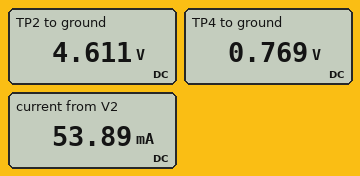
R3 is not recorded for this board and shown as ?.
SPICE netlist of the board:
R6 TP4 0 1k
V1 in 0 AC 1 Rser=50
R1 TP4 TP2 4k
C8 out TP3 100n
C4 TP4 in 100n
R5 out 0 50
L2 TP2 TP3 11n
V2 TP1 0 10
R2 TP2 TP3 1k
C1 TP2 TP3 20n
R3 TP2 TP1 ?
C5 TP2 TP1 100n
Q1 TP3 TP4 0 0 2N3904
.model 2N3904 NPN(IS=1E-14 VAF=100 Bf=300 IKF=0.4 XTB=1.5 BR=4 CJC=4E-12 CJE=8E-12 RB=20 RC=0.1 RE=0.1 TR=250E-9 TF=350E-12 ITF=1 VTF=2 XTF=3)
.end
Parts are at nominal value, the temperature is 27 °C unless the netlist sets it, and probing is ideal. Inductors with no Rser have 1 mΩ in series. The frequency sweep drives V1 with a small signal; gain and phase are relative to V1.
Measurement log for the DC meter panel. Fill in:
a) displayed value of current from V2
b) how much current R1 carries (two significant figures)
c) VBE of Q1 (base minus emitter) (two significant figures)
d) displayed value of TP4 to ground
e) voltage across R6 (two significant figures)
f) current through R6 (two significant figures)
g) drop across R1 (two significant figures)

53.89 mA
960 µA
770 mV
0.769 V
770 mV
770 µA
3.8 V
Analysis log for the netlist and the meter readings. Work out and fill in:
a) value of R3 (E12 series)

100 Ω
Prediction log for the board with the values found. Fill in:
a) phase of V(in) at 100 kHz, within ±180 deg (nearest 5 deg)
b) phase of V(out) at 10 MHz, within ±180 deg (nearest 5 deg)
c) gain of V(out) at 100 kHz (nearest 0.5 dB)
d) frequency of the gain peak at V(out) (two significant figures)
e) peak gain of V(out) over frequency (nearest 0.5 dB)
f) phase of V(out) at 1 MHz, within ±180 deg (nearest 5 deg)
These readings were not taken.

5 deg
-155 deg
22.0 dB
11 MHz
25.0 dB
85 deg
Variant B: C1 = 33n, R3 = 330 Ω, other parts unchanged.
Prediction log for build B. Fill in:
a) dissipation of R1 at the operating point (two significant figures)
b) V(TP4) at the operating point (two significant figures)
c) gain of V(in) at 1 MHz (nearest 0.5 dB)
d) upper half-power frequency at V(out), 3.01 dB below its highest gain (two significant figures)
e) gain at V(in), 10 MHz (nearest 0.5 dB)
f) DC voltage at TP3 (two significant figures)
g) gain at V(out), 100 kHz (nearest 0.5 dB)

2.5 mW
730 mV
-1.5 dB
8.4 MHz
-3.5 dB
3.9 V
16.5 dB
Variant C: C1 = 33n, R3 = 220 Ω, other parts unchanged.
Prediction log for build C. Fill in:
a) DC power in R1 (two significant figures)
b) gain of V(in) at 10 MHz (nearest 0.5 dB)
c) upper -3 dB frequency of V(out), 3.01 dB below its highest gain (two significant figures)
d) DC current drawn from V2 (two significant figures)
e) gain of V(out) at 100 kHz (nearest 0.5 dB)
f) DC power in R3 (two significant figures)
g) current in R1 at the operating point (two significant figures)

2.8 mW
-4.5 dB
8.4 MHz
27 mA
19.0 dB
160 mW
830 µA
